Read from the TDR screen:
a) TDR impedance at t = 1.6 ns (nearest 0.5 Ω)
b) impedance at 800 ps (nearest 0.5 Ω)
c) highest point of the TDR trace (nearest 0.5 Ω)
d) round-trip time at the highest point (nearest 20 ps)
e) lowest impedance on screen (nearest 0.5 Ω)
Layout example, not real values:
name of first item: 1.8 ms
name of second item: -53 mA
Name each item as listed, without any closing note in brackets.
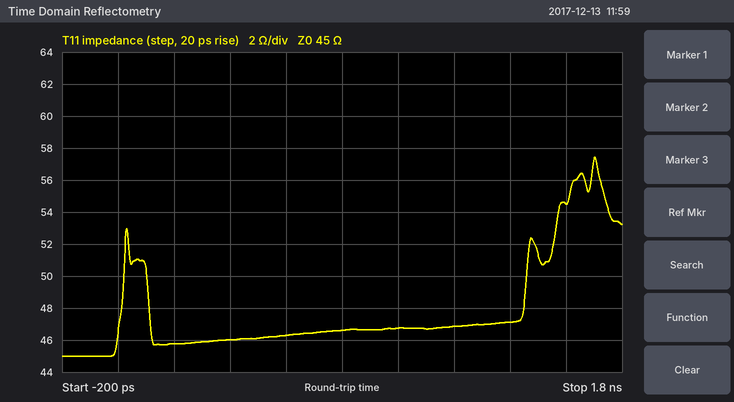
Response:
TDR impedance at t = 1.6 ns: 54.5 Ω
impedance at 800 ps: 46.5 Ω
highest point of the TDR trace: 57.5 Ω
round-trip time at the highest point: 1.70 ns
lowest impedance on screen: 45.0 Ω
